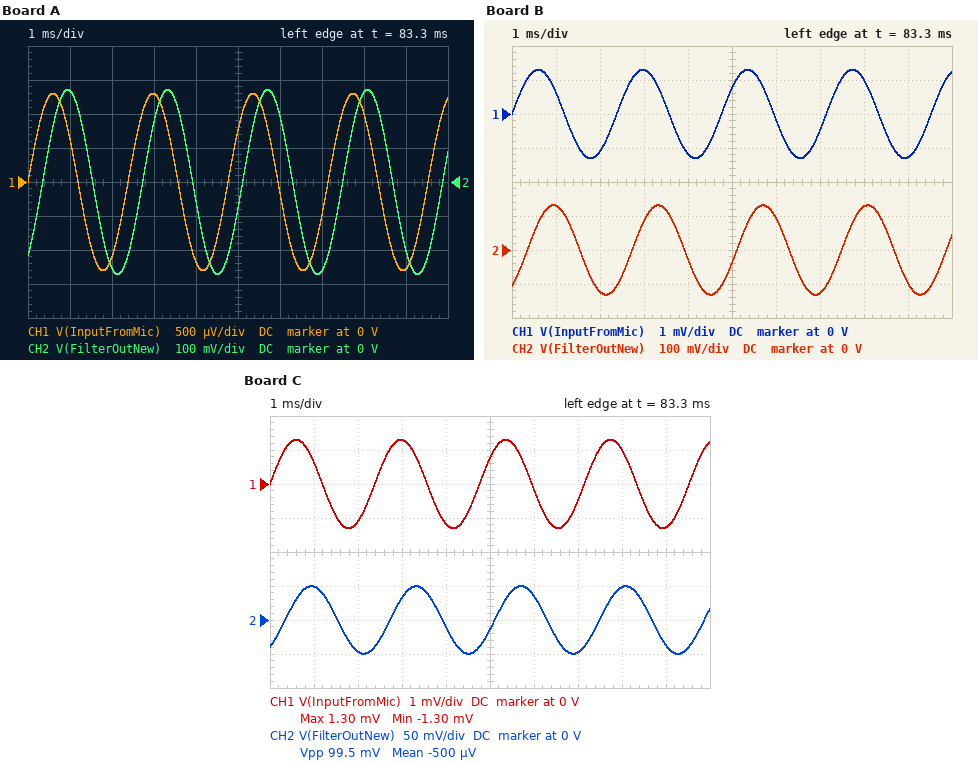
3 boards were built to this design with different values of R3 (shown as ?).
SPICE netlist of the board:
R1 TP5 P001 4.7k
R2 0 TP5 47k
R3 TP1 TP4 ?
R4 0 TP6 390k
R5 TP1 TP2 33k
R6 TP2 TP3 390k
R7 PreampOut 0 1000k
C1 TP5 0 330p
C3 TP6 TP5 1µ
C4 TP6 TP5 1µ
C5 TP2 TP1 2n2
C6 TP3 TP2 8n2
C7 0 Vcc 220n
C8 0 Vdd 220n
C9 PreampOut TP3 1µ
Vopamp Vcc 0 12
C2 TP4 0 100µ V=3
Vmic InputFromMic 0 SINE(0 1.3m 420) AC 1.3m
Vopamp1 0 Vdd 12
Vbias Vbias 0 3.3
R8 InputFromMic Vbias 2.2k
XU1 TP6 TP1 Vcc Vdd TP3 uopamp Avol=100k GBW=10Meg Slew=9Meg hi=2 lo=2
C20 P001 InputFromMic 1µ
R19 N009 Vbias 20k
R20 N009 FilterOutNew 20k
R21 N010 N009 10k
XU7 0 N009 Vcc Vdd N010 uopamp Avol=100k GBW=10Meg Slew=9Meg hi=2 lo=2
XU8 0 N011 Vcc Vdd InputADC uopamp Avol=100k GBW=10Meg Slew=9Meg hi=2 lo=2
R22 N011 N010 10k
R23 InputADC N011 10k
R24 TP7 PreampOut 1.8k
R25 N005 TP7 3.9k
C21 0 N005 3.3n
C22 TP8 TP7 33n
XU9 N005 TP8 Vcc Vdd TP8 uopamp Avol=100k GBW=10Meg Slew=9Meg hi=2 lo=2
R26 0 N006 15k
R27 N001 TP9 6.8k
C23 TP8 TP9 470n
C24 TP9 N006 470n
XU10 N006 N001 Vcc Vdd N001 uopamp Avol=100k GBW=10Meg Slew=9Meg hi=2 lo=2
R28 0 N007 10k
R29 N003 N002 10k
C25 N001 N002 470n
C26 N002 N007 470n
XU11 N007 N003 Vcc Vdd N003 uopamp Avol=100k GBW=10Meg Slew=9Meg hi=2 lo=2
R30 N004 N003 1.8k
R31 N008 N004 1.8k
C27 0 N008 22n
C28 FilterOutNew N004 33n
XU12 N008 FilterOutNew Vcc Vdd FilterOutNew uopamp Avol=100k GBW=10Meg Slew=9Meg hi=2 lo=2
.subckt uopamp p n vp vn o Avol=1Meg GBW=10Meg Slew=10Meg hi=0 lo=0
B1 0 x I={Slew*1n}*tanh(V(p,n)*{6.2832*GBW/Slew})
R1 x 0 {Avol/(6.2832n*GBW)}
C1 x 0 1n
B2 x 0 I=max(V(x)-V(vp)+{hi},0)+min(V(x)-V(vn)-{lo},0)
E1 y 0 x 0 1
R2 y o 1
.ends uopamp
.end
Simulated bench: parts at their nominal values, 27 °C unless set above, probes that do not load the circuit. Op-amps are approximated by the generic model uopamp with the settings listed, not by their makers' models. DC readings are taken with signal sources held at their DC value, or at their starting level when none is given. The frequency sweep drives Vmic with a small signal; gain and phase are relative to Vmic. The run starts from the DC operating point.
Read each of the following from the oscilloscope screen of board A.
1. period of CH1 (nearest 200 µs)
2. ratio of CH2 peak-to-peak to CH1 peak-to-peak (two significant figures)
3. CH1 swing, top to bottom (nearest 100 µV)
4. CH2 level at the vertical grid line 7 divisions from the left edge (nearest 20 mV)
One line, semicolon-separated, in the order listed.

2.4 ms; 210; 2.6 mV; -260 mV
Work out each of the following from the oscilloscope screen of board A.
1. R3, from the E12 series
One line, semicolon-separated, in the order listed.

270 Ω
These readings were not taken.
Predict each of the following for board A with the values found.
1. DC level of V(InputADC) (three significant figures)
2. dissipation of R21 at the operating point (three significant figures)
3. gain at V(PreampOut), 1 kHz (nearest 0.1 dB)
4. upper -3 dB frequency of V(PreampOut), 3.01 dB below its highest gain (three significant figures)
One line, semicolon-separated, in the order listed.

1.65 V; 272 µW; 42.9 dB; 63.2 Hz
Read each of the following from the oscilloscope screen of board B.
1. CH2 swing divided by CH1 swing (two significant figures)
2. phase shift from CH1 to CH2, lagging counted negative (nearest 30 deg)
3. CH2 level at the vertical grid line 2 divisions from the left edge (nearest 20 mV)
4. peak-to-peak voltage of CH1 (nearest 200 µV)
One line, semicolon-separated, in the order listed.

100; -60 deg; -120 mV; 2.6 mV
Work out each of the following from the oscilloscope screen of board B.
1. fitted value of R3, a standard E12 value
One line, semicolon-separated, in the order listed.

560 Ω
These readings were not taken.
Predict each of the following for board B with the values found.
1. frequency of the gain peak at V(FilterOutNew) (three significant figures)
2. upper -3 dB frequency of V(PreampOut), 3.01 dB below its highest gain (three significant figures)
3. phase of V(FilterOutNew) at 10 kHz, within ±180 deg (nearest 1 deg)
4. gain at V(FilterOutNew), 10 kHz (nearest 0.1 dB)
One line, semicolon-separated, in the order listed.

61.5 Hz; 58.9 Hz; -20 deg; -4.0 dB
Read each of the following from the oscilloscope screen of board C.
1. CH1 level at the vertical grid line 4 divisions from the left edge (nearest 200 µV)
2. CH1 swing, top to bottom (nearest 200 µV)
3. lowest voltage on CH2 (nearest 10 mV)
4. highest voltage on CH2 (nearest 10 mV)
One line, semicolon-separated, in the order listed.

-1.2 mV; 2.6 mV; -50 mV; 50 mV
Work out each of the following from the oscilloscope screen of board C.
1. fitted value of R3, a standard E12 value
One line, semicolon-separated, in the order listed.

1.5 kΩ
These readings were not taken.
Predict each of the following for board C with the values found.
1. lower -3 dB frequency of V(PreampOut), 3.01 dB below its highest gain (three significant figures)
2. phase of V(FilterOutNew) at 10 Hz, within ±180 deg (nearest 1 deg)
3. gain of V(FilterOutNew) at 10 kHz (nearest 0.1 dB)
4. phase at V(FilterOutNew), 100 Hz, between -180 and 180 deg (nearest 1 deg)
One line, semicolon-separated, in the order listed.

3.32 Hz; -41 deg; -12.3 dB; 9 deg
